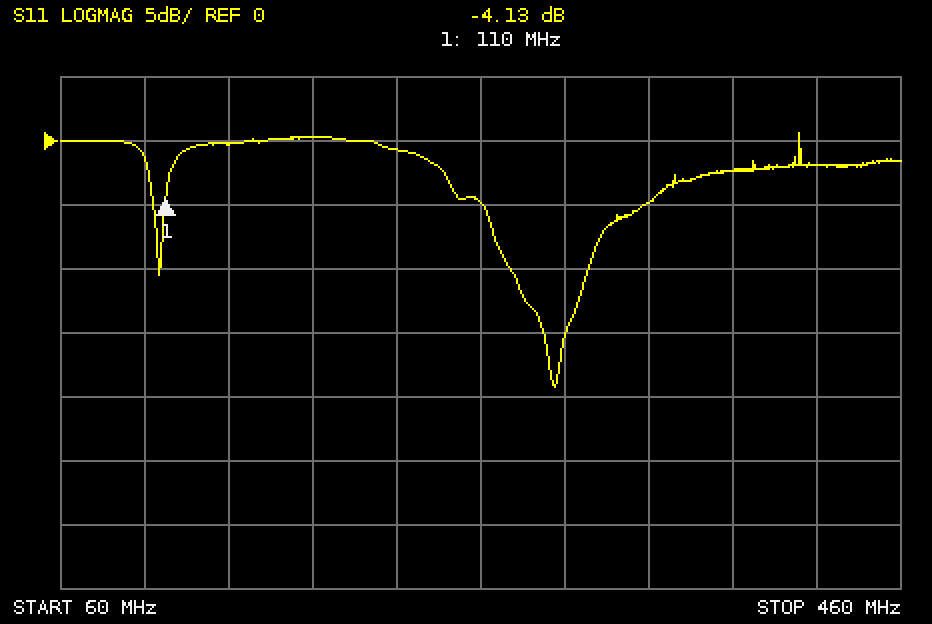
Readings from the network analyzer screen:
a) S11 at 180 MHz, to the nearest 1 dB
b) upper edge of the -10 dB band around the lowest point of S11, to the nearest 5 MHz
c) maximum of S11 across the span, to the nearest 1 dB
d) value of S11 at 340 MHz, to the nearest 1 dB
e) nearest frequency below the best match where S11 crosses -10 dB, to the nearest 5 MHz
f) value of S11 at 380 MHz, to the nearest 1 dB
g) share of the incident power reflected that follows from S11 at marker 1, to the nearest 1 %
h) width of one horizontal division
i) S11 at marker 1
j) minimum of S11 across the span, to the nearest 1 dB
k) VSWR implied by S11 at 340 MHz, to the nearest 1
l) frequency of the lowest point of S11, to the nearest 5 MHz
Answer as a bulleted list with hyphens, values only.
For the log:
- 0 dB
- 310 MHz
- 1 dB
- -5 dB
- 275 MHz
- -2 dB
- 39 %
- 40 MHz
- -4.13 dB
- -19 dB
- 4
- 295 MHz
